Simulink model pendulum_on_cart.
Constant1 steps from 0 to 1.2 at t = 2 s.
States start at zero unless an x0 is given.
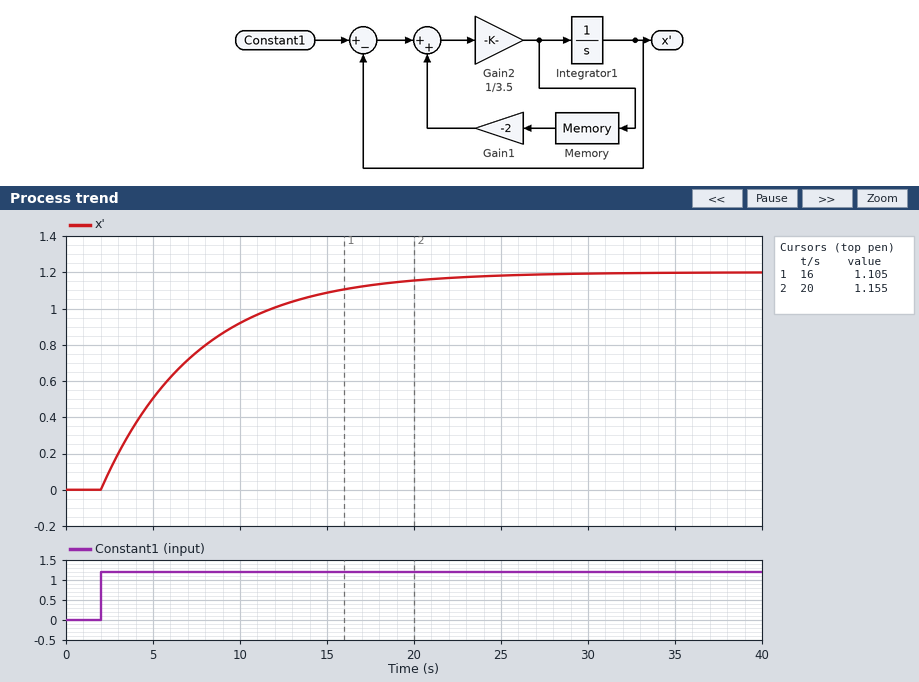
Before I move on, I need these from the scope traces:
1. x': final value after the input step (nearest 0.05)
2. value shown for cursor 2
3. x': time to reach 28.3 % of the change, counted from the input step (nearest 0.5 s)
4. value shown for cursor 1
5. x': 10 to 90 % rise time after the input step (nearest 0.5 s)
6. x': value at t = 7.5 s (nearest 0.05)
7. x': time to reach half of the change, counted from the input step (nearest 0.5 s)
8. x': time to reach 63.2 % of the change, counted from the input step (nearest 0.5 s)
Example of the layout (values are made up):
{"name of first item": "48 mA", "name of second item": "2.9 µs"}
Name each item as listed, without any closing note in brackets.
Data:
{"x': final value after the input step": "1.20", "value shown for cursor 2": "1.155", "x': time to reach 28.3 % of the change, counted from the input step": "2.0 s", "value shown for cursor 1": "1.105", "x': 10 to 90 % rise time after the input step": "12.0 s", "x': value at t = 7.5 s": "0.75", "x': time to reach half of the change, counted from the input step": "4.0 s", "x': time to reach 63.2 % of the change, counted from the input step": "5.5 s"}
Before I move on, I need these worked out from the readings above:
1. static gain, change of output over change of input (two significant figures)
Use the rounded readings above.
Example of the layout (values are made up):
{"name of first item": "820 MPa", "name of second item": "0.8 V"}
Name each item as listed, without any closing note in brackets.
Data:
{"static gain, change of output over change of input": "1.0"}
